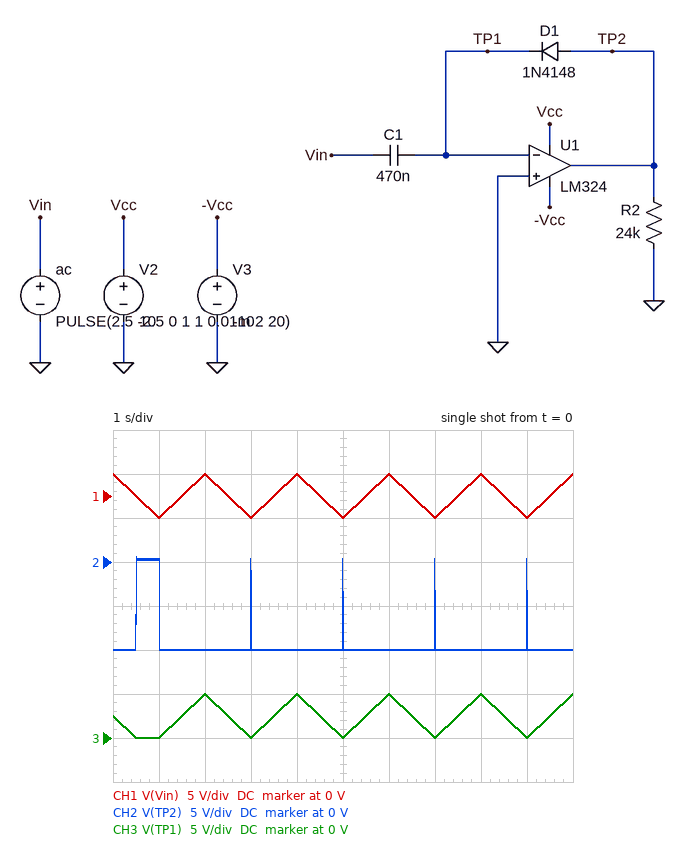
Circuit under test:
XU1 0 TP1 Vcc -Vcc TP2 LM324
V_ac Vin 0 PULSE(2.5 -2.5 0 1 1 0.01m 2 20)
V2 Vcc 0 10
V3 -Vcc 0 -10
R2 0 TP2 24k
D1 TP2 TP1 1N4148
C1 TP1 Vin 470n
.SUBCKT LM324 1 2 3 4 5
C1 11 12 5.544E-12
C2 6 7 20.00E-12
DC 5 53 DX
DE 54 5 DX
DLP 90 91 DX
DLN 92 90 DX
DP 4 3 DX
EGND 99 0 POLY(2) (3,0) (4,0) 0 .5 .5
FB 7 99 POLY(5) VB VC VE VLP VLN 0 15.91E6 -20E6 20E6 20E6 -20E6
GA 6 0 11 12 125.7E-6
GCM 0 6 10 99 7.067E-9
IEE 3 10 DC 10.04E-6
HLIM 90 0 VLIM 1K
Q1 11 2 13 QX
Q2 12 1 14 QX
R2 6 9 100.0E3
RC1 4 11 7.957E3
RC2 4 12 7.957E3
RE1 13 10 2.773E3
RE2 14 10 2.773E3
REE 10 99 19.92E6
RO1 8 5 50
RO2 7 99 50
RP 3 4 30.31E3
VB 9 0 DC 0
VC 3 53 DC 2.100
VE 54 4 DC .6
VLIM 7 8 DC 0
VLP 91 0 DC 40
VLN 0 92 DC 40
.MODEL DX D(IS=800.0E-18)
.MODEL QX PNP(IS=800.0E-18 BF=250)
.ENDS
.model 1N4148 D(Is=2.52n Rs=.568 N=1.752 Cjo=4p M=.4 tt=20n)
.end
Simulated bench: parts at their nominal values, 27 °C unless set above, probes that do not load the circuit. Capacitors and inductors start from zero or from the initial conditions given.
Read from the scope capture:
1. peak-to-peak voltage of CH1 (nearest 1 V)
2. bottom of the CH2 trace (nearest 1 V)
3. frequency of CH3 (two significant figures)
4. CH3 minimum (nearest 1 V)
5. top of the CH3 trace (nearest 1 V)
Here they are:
5 V
-10 V
500 mHz
0 V
5 V
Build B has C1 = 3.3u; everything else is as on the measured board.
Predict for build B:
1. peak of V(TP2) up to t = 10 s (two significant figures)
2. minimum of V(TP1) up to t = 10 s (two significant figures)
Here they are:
610 mV
-4.0 mV
